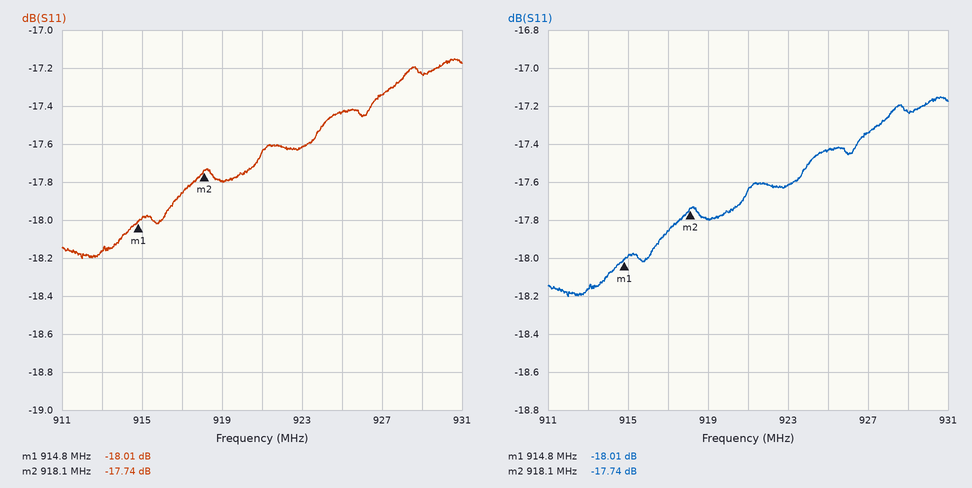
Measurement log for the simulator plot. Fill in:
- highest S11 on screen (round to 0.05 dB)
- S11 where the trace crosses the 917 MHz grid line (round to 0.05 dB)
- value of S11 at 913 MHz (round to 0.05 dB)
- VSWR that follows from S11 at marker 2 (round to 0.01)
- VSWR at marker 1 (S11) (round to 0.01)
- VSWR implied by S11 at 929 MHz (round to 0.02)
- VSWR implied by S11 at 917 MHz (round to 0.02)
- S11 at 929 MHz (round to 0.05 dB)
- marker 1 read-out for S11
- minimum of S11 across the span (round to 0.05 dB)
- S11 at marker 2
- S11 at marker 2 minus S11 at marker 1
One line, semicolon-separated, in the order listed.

-17.15 dB; -17.85 dB; -18.15 dB; 1.30; 1.29; 1.32; 1.30; -17.25 dB; -18.01 dB; -18.20 dB; -17.74 dB; 0.27 dB
